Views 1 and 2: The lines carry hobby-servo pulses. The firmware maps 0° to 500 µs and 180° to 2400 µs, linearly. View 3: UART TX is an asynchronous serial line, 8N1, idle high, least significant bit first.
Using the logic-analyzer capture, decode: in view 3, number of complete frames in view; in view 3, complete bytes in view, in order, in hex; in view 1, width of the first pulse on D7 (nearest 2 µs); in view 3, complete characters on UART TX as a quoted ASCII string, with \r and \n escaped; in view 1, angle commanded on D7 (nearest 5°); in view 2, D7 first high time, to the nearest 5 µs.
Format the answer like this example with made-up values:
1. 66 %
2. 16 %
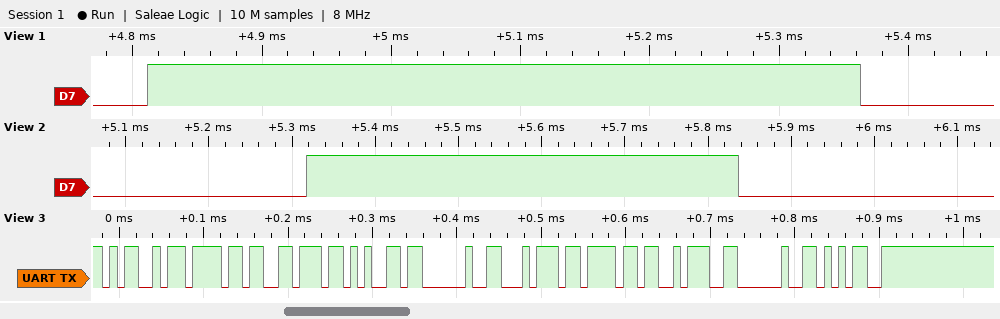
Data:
1. 10
2. 4D 6F 76 65 20 74 6F 3A 20 35
3. 552 µs
4. "Move to: 5"
5. 5°
6. 520 µs
